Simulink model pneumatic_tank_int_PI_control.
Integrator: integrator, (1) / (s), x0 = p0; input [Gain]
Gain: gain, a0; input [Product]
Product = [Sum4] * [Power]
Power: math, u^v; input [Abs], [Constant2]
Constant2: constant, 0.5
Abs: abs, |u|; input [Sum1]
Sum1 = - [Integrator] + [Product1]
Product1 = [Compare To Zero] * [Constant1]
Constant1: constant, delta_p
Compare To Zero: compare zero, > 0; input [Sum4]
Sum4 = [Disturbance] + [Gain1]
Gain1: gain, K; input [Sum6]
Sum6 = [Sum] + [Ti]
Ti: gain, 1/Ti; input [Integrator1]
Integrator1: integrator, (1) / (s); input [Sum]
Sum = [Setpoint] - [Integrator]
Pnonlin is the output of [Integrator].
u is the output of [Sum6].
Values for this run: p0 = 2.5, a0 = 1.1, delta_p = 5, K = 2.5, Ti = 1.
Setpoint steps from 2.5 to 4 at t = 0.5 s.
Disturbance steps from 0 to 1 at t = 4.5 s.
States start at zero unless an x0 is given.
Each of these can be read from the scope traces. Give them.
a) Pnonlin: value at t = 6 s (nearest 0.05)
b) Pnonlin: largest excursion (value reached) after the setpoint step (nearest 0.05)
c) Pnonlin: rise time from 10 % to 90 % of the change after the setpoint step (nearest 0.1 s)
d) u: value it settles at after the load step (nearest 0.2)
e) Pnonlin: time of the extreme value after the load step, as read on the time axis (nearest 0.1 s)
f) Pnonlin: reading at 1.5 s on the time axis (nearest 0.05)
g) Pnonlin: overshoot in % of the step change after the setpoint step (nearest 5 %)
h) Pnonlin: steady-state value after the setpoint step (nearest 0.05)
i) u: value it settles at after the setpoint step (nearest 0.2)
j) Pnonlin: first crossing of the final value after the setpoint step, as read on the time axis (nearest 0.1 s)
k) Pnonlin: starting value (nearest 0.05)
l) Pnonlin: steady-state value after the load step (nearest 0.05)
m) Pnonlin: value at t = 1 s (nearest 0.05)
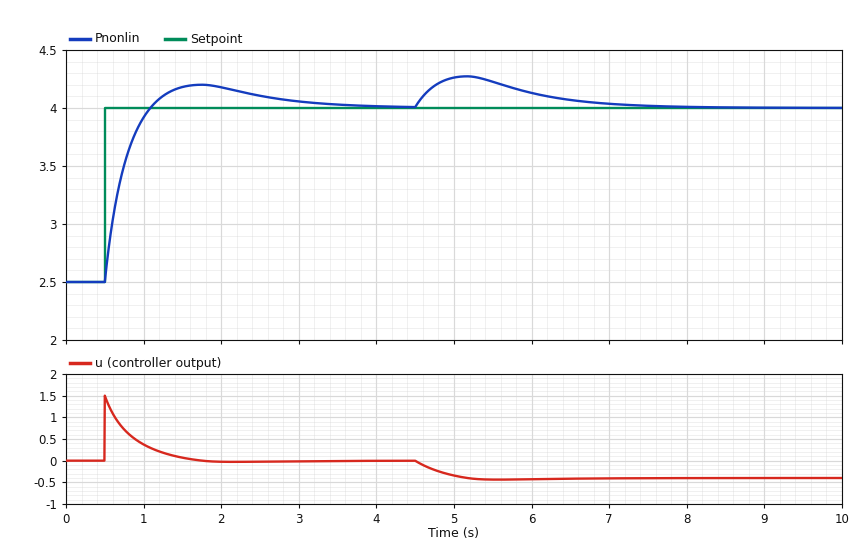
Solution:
4.15
4.20
0.4 s
-0.4
5.2 s
4.20
15 %
4.00
0.0
1.1 s
2.50
4.00
3.90
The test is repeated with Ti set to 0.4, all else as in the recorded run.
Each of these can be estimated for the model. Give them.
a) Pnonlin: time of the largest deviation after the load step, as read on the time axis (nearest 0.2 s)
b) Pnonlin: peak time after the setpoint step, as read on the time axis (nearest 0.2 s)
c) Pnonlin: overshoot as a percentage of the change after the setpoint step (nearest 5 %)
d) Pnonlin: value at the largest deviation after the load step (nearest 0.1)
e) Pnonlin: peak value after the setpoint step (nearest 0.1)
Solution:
5.0 s
1.4 s
20 %
4.2
4.3
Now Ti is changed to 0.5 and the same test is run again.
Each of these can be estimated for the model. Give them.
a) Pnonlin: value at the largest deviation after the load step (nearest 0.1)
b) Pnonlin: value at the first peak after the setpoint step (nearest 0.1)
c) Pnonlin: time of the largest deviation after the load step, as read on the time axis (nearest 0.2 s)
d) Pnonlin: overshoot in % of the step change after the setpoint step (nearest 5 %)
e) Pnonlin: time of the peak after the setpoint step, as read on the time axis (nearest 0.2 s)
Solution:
4.2
4.3
5.0 s
20 %
1.4 s
